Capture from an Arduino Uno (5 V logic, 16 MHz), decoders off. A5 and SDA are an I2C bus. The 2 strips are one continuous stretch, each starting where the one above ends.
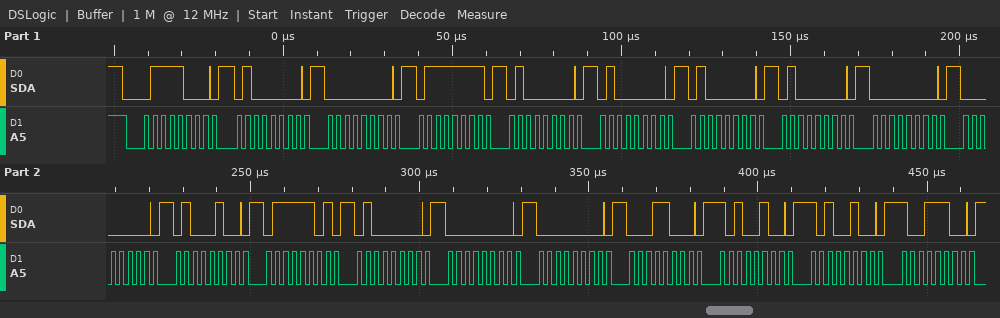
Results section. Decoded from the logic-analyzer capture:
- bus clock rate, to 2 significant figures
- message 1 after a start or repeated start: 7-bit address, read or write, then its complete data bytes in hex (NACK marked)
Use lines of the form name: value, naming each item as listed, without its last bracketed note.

bus clock rate, to 2 significant figures: 400 kHz
message 1 after a start or repeated start: 7-bit address, read or write, then its complete data bytes in hex: 0x3C write: 40 00 7F 40 40 40 40 00 00 44 7D 40 00 00 18 A4 A4 9C
